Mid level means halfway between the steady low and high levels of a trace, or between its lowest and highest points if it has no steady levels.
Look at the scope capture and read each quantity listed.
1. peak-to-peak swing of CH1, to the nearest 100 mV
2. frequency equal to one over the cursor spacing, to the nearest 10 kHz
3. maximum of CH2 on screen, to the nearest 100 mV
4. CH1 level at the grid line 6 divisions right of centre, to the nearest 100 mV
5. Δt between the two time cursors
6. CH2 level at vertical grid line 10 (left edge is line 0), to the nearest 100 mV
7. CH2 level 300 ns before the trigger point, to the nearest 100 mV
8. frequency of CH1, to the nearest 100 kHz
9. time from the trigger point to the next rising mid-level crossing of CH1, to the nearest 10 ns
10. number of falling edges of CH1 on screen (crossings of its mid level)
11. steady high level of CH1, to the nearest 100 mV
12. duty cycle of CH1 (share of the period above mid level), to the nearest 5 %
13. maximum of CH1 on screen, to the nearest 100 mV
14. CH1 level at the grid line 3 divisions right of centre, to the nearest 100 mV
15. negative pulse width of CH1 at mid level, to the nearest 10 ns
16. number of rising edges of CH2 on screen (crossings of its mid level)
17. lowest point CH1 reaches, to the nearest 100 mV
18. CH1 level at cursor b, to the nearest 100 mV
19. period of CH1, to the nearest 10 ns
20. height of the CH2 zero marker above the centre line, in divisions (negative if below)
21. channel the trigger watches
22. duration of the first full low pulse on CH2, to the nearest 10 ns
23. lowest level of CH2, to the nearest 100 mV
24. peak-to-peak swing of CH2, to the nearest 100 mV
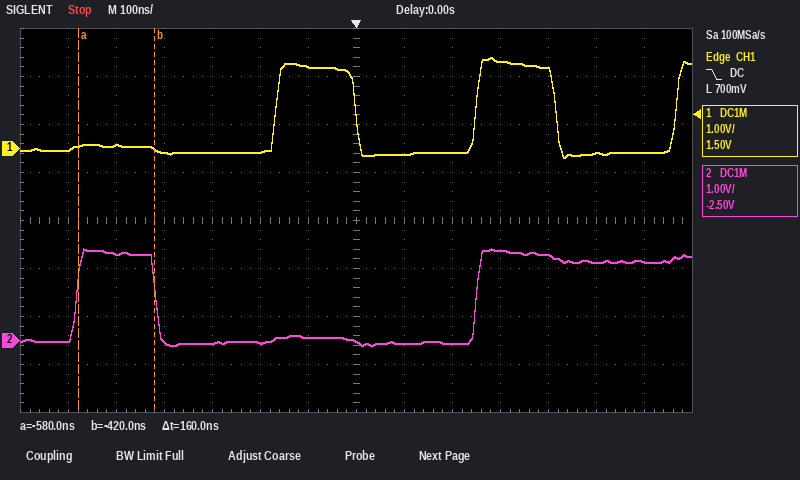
2.1 V
6.25 MHz
1.9 V
-100 mV
160 ns
1.9 V
-100 mV
2.4 MHz
250 ns
2
1.7 V
40 %
1.9 V
1.8 V
250 ns
2
-200 mV
0.0 V
420 ns
-2.5 div
CH1
670 ns
-100 mV
2.0 V
